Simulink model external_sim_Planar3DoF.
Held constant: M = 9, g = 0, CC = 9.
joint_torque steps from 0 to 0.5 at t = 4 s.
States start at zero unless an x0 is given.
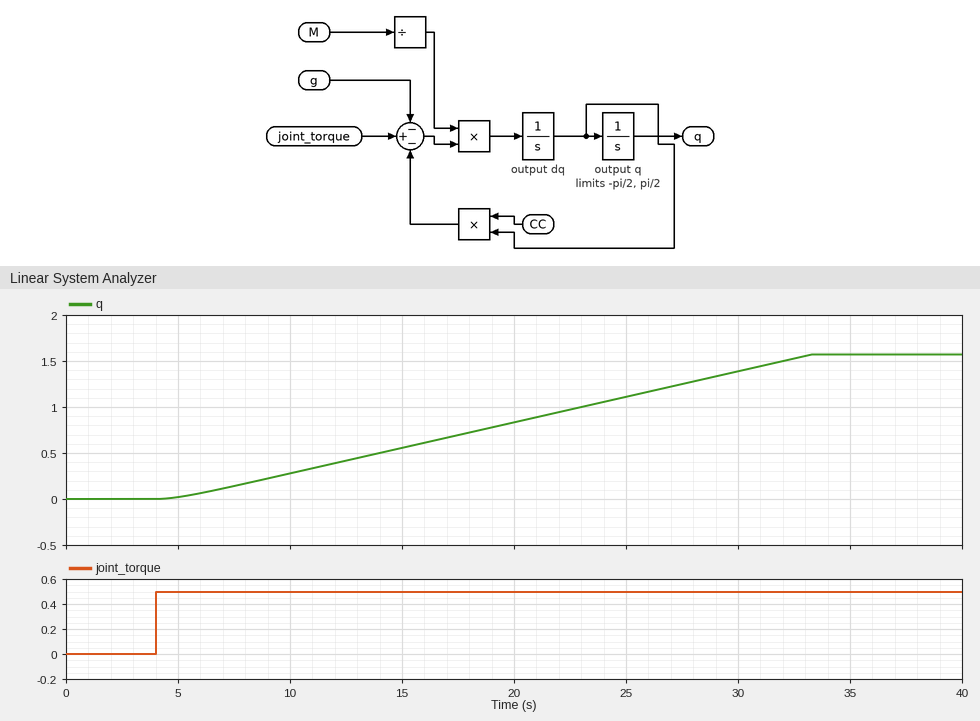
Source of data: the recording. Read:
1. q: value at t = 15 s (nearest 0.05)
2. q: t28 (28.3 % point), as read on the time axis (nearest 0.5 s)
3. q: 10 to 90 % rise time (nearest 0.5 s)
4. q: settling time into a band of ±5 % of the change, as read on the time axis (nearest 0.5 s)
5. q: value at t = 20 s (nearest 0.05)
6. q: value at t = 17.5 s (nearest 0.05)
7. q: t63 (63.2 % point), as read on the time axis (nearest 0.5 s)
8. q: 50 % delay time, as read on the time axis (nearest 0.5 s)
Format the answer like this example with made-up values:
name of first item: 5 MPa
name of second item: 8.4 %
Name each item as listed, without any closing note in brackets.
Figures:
q: value at t = 15 s: 0.55
q: t28 (28.3 % point), as read on the time axis: 13.0 s
q: 10 to 90 % rise time: 22.5 s
q: settling time into a band of ±5 % of the change, as read on the time axis: 32.0 s
q: value at t = 20 s: 0.85
q: value at t = 17.5 s: 0.70
q: t63 (63.2 % point), as read on the time axis: 23.0 s
q: 50 % delay time, as read on the time axis: 19.0 s
